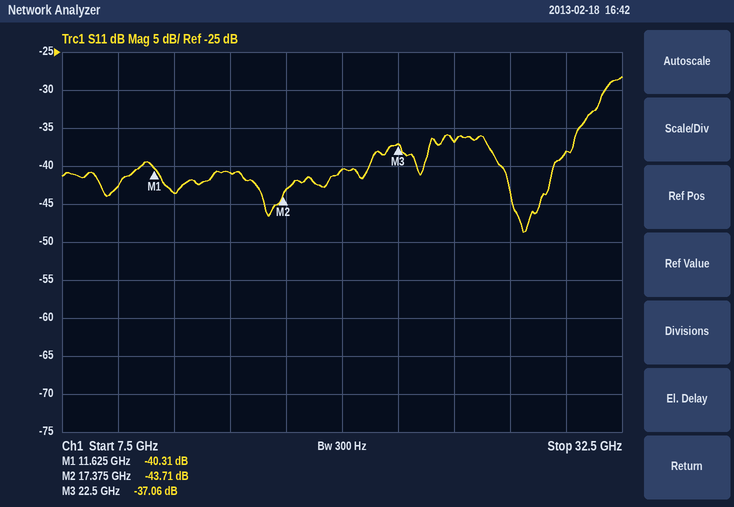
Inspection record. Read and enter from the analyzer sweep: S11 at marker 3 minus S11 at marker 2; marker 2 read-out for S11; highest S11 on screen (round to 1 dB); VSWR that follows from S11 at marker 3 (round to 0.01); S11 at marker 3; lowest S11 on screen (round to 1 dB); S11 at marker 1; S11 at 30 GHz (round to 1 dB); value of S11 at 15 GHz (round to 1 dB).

6.65 dB
-43.71 dB
-28 dB
1.03
-37.06 dB
-49 dB
-40.31 dB
-38 dB
-41 dB
